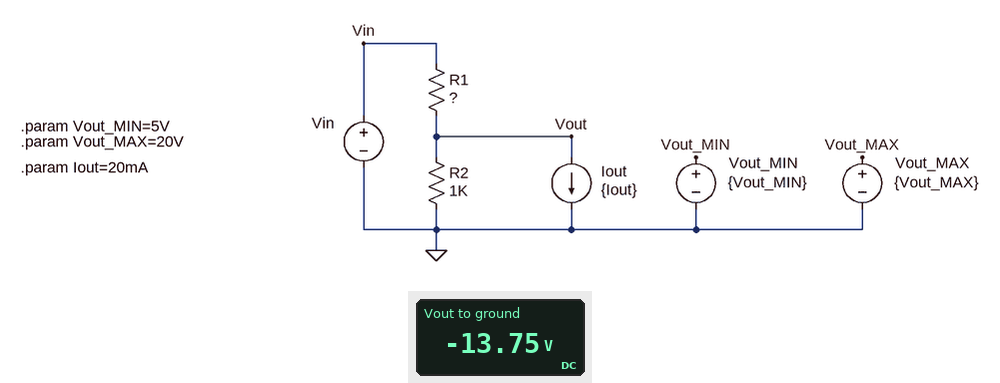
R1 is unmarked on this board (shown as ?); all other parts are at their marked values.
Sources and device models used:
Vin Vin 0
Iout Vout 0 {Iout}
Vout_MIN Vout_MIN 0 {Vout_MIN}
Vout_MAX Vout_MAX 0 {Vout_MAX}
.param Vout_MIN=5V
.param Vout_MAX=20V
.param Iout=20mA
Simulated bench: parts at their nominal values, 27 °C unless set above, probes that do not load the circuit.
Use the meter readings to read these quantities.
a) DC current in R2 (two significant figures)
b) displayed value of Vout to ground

14 mA
-13.75 V
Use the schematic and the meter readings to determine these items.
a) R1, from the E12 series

2.2 kΩ
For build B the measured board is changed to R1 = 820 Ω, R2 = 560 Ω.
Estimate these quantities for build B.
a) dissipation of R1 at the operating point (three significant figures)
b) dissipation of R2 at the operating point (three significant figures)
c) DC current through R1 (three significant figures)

54.0 mW
79.1 mW
8.12 mA
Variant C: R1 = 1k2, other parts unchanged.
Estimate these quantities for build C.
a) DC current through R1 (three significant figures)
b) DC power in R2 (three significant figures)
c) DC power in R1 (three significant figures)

9.09 mA
119 mW
99.2 mW
